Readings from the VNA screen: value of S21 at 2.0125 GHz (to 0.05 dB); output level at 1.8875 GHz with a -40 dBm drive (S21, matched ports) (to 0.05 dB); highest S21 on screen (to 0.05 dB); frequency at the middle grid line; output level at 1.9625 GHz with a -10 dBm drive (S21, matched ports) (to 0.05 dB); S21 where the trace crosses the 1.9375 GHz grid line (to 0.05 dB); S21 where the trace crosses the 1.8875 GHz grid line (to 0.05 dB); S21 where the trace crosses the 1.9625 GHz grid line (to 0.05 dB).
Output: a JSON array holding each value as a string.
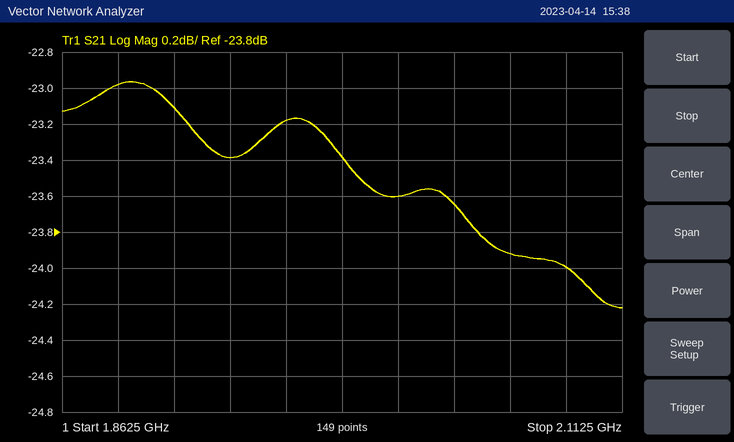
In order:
["-23.60 dB", "-63.00 dBm", "-22.95 dB", "1.9875 GHz", "-33.20 dBm", "-23.40 dB", "-23.00 dB", "-23.20 dB"]
